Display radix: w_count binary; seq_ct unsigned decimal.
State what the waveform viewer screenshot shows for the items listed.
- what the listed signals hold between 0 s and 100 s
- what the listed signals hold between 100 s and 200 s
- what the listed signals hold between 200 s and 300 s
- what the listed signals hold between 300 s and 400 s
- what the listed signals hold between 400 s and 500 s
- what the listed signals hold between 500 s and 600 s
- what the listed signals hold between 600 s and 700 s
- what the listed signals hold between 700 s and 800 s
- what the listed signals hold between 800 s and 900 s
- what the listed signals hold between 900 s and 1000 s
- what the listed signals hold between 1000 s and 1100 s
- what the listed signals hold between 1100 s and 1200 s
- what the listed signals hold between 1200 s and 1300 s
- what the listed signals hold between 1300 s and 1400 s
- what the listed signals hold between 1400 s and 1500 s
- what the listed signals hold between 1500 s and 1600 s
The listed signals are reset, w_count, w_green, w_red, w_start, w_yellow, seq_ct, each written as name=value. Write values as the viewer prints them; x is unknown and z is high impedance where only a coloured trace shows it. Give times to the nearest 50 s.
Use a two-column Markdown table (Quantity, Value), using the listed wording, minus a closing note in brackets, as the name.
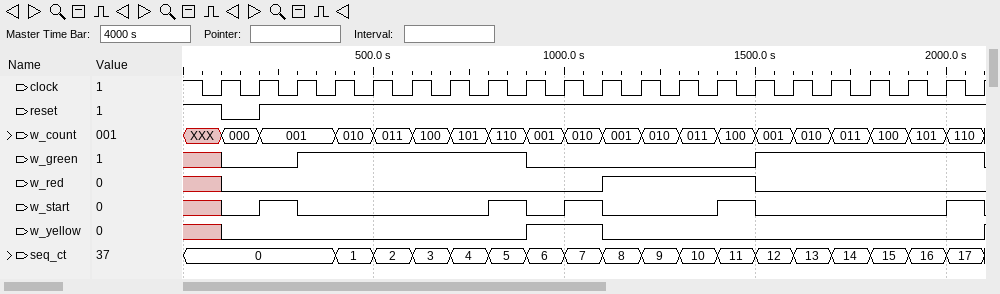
| Quantity | Value |
|---|---|
| what the listed signals hold between 0 s and 100 s | reset=1, w_count=XXX, w_green=x, w_red=x, w_start=x, w_yellow=x, seq_ct=0 |
| what the listed signals hold between 100 s and 200 s | reset=0, w_count=000, w_green=0, w_red=0, w_start=0, w_yellow=0, seq_ct=0 |
| what the listed signals hold between 200 s and 300 s | reset=1, w_count=001, w_green=0, w_red=0, w_start=1, w_yellow=0, seq_ct=0 |
| what the listed signals hold between 300 s and 400 s | reset=1, w_count=001, w_green=1, w_red=0, w_start=0, w_yellow=0, seq_ct=0 |
| what the listed signals hold between 400 s and 500 s | reset=1, w_count=010, w_green=1, w_red=0, w_start=0, w_yellow=0, seq_ct=1 |
| what the listed signals hold between 500 s and 600 s | reset=1, w_count=011, w_green=1, w_red=0, w_start=0, w_yellow=0, seq_ct=2 |
| what the listed signals hold between 600 s and 700 s | reset=1, w_count=100, w_green=1, w_red=0, w_start=0, w_yellow=0, seq_ct=3 |
| what the listed signals hold between 700 s and 800 s | reset=1, w_count=101, w_green=1, w_red=0, w_start=0, w_yellow=0, seq_ct=4 |
| what the listed signals hold between 800 s and 900 s | reset=1, w_count=110, w_green=1, w_red=0, w_start=1, w_yellow=0, seq_ct=5 |
| what the listed signals hold between 900 s and 1000 s | reset=1, w_count=001, w_green=0, w_red=0, w_start=0, w_yellow=1, seq_ct=6 |
| what the listed signals hold between 1000 s and 1100 s | reset=1, w_count=010, w_green=0, w_red=0, w_start=1, w_yellow=1, seq_ct=7 |
| what the listed signals hold between 1100 s and 1200 s | reset=1, w_count=001, w_green=0, w_red=1, w_start=0, w_yellow=0, seq_ct=8 |
| what the listed signals hold between 1200 s and 1300 s | reset=1, w_count=010, w_green=0, w_red=1, w_start=0, w_yellow=0, seq_ct=9 |
| what the listed signals hold between 1300 s and 1400 s | reset=1, w_count=011, w_green=0, w_red=1, w_start=0, w_yellow=0, seq_ct=10 |
| what the listed signals hold between 1400 s and 1500 s | reset=1, w_count=100, w_green=0, w_red=1, w_start=1, w_yellow=0, seq_ct=11 |
| what the listed signals hold between 1500 s and 1600 s | reset=1, w_count=001, w_green=1, w_red=0, w_start=0, w_yellow=0, seq_ct=12 |
